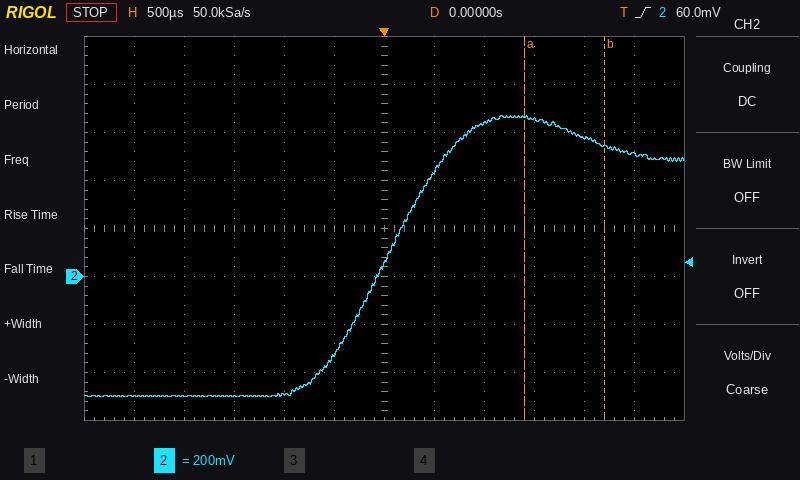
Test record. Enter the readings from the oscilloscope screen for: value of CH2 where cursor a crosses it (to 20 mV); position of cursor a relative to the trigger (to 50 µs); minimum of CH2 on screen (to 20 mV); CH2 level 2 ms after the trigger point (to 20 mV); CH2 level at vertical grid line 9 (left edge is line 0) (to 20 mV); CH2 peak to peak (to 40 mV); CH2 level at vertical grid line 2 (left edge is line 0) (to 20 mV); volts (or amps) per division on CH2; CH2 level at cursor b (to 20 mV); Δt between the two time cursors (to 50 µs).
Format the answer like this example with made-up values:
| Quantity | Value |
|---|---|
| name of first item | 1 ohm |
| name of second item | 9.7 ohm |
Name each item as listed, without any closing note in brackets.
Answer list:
| Quantity | Value |
|---|---|
| value of CH2 where cursor a crosses it | 660 mV |
| position of cursor a relative to the trigger | +1.40 ms |
| minimum of CH2 on screen | -500 mV |
| CH2 level 2 ms after the trigger point | 580 mV |
| CH2 level at vertical grid line 9 (left edge is line 0) | 660 mV |
| CH2 peak to peak | 1.16 V |
| CH2 level at vertical grid line 2 (left edge is line 0) | -500 mV |
| volts (or amps) per division on CH2 | 200 mV |
| CH2 level at cursor b | 540 mV |
| Δt between the two time cursors | 800 µs |
